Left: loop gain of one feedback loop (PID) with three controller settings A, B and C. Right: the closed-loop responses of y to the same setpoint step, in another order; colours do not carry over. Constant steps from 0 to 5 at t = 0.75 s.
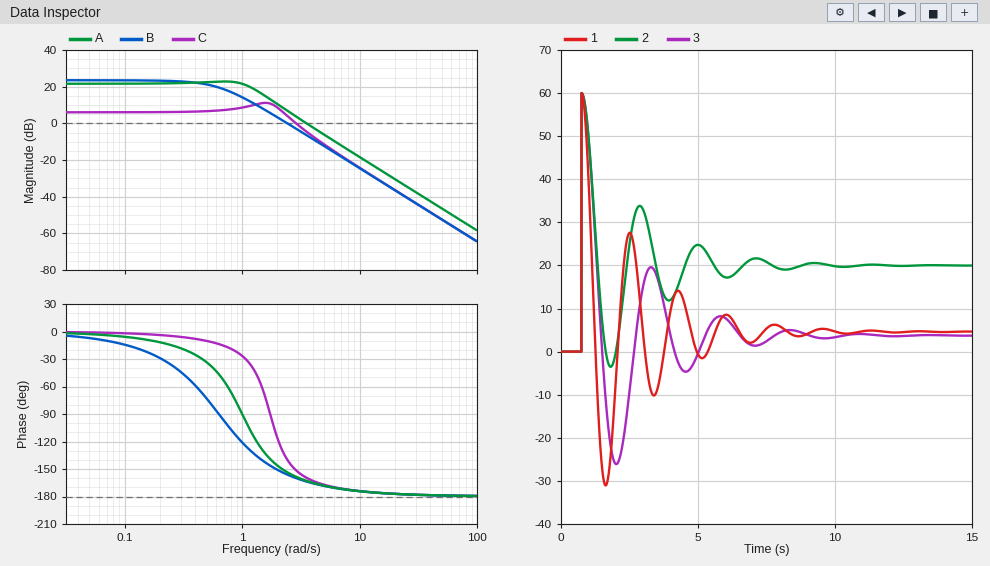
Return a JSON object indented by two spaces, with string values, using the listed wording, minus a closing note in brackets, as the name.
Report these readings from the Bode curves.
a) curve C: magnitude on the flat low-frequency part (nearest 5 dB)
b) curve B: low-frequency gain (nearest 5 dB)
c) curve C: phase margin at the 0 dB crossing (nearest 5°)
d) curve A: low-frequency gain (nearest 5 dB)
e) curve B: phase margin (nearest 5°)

{
  "curve C: magnitude on the flat low-frequency part": "5 dB",
  "curve B: low-frequency gain": "25 dB",
  "curve C: phase margin at the 0 dB crossing": "30°",
  "curve A: low-frequency gain": "20 dB",
  "curve B: phase margin": "25°"
}
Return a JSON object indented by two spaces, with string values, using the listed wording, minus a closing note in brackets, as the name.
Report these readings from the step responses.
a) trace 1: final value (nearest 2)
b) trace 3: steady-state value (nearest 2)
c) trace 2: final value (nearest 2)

{
  "trace 1: final value": "4",
  "trace 3: steady-state value": "4",
  "trace 2: final value": "20"
}
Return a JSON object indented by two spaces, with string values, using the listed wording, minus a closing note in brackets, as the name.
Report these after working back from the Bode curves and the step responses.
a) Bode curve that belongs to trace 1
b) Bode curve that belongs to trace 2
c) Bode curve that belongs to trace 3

{
  "Bode curve that belongs to trace 1": "A",
  "Bode curve that belongs to trace 2": "C",
  "Bode curve that belongs to trace 3": "B"
}
